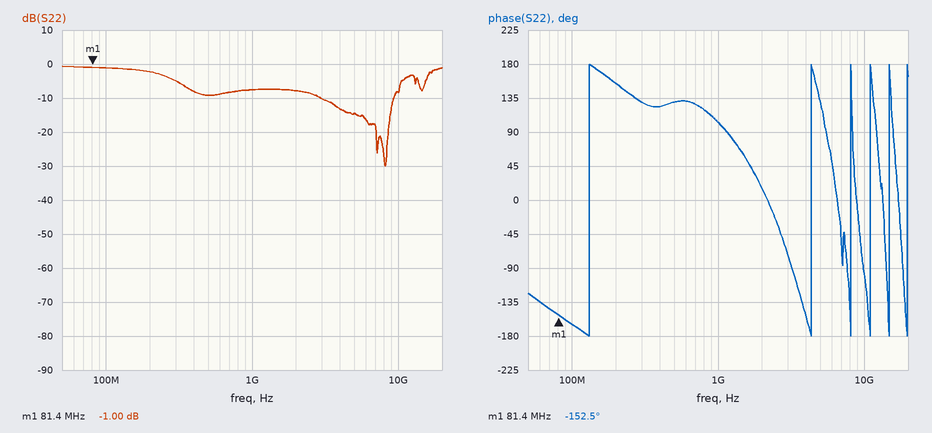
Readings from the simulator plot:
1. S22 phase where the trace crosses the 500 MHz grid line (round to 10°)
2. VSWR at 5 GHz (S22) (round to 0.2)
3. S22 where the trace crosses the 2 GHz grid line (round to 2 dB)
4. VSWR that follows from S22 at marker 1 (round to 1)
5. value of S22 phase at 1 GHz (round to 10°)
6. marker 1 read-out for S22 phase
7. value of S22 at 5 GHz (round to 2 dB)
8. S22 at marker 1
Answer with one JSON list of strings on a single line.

["130°", "1.4", "-8 dB", "17", "100°", "-152.5°", "-14 dB", "-1.00 dB"]
